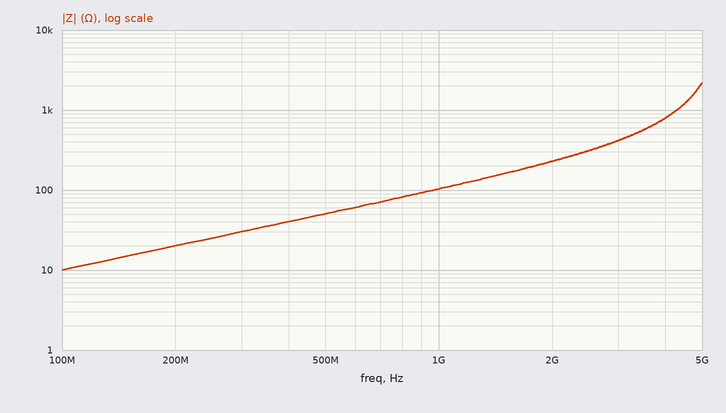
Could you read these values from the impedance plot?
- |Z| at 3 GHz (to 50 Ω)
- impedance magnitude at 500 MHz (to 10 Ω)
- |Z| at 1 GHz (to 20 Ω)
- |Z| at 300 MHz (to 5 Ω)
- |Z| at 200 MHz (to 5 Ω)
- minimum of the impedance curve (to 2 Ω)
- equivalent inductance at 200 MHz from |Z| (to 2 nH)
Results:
400 Ω
50 Ω
100 Ω
30 Ω
20 Ω
10 Ω
16 nH
